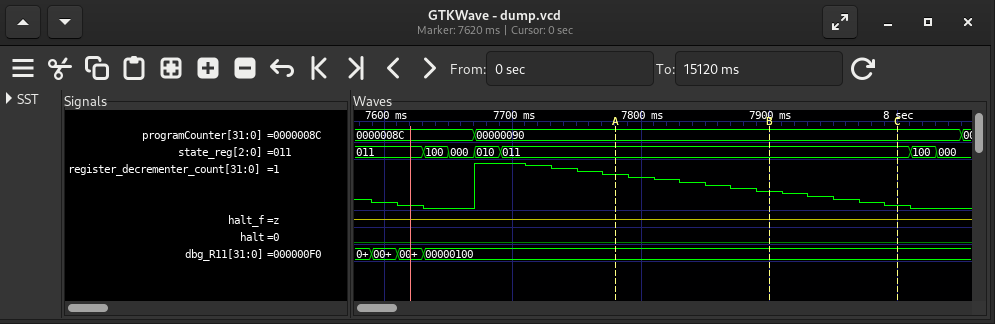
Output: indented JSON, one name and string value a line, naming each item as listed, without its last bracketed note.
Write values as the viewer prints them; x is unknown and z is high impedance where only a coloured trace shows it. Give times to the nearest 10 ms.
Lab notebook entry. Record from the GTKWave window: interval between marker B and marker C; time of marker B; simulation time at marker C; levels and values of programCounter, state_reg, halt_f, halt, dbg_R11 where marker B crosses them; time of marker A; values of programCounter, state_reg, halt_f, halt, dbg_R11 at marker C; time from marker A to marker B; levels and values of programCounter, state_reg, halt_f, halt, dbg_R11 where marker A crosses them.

{
  "interval between marker B and marker C": "100 ms",
  "time of marker B": "7900 ms",
  "simulation time at marker C": "8000 ms",
  "levels and values of programCounter, state_reg, halt_f, halt, dbg_R11 where marker B crosses them": "programCounter=00000090, state_reg=011, halt_f=z, halt=0, dbg_R11=00000100",
  "time of marker A": "7780 ms",
  "values of programCounter, state_reg, halt_f, halt, dbg_R11 at marker C": "programCounter=00000090, state_reg=011, halt_f=z, halt=0, dbg_R11=00000100",
  "time from marker A to marker B": "120 ms",
  "levels and values of programCounter, state_reg, halt_f, halt, dbg_R11 where marker A crosses them": "programCounter=00000090, state_reg=011, halt_f=z, halt=0, dbg_R11=00000100"
}
